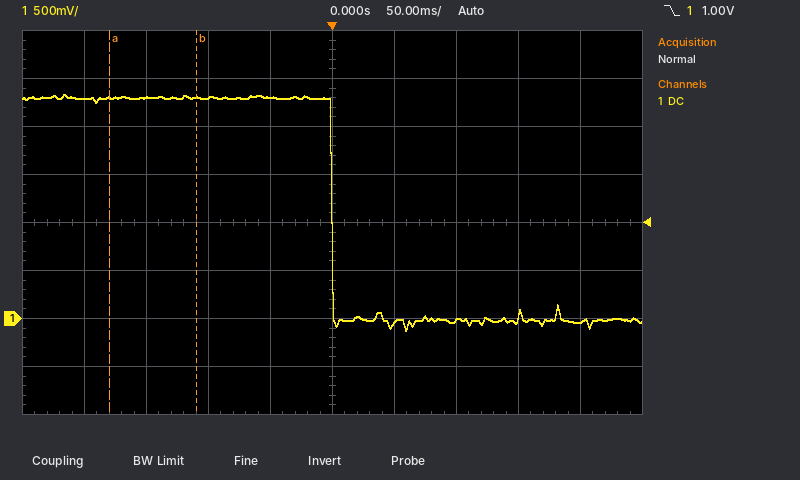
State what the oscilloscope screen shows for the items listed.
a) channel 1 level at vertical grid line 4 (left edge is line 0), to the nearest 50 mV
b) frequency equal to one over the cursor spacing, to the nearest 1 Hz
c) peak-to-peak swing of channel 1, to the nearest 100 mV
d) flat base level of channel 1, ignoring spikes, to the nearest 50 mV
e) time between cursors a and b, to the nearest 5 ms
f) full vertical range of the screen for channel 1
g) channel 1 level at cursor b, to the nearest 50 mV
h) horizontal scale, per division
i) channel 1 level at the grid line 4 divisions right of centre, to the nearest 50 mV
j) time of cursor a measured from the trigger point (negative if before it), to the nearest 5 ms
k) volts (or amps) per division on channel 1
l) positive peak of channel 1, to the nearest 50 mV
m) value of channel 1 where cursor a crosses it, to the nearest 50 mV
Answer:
2.30 V
14 Hz
2.50 V
0 mV
70 ms
4 V
2.30 V
50 ms
-50 mV
-180 ms
500 mV
2.35 V
2.30 V
